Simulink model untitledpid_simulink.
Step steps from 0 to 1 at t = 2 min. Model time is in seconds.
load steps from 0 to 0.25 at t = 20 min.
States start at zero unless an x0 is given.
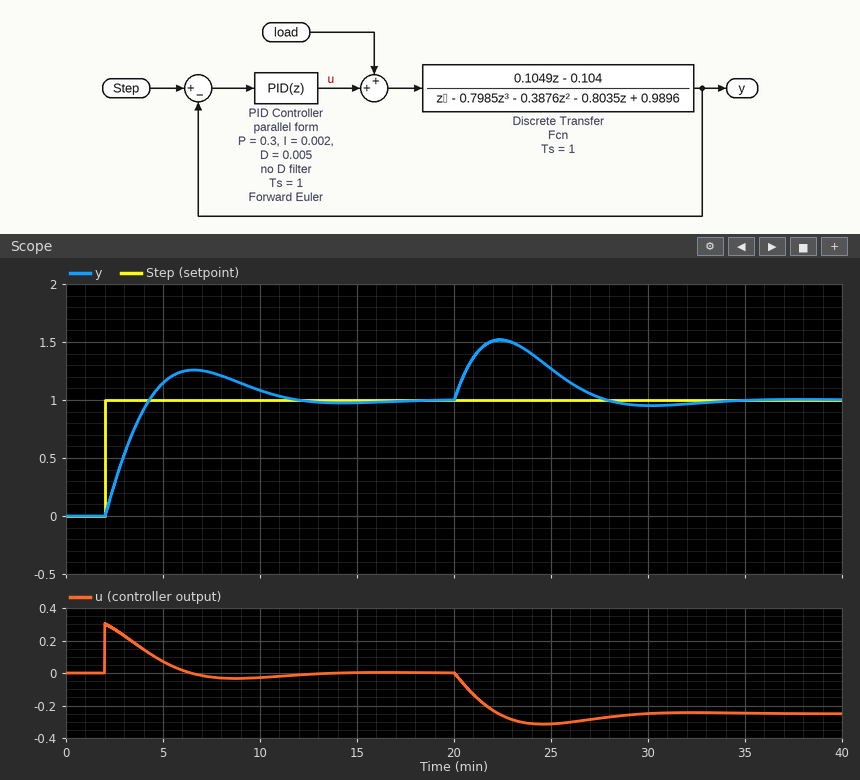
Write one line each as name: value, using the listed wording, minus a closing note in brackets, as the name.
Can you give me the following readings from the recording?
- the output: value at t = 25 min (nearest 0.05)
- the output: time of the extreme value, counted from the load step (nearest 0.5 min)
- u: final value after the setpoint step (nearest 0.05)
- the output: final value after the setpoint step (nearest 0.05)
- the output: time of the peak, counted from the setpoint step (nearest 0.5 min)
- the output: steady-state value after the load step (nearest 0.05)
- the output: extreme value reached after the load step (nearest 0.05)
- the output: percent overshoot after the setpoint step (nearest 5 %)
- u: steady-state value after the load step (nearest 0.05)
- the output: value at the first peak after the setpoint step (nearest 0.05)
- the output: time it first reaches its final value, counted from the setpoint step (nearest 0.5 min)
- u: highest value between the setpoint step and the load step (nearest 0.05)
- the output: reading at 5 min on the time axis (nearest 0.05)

the output: value at t = 25 min: 1.25
the output: time of the extreme value, counted from the load step: 2.5 min
u: final value after the setpoint step: 0.00
the output: final value after the setpoint step: 1.00
the output: time of the peak, counted from the setpoint step: 4.5 min
the output: steady-state value after the load step: 1.00
the output: extreme value reached after the load step: 1.50
the output: percent overshoot after the setpoint step: 25 %
u: steady-state value after the load step: -0.25
the output: value at the first peak after the setpoint step: 1.25
the output: time it first reaches its final value, counted from the setpoint step: 2.5 min
u: highest value between the setpoint step and the load step: 0.30
the output: reading at 5 min on the time axis: 1.15
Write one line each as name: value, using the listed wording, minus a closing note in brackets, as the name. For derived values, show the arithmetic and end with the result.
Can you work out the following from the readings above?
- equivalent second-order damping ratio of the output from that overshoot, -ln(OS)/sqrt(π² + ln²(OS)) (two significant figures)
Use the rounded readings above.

equivalent second-order damping ratio of the output from that overshoot, -ln(OS)/sqrt(π² + ln²(OS)): ln(0.25) = -1.386; 1.386 / sqrt(9.870 + 1.922) = 0.40
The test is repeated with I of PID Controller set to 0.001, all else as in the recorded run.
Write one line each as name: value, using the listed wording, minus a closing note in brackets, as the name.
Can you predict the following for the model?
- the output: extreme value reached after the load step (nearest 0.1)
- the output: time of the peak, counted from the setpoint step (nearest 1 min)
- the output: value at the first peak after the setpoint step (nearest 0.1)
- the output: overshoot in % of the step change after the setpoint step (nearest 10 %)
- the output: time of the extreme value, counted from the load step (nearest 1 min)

the output: extreme value reached after the load step: 1.6
the output: time of the peak, counted from the setpoint step: 6 min
the output: value at the first peak after the setpoint step: 1.2
the output: overshoot in % of the step change after the setpoint step: 20 %
the output: time of the extreme value, counted from the load step: 3 min
